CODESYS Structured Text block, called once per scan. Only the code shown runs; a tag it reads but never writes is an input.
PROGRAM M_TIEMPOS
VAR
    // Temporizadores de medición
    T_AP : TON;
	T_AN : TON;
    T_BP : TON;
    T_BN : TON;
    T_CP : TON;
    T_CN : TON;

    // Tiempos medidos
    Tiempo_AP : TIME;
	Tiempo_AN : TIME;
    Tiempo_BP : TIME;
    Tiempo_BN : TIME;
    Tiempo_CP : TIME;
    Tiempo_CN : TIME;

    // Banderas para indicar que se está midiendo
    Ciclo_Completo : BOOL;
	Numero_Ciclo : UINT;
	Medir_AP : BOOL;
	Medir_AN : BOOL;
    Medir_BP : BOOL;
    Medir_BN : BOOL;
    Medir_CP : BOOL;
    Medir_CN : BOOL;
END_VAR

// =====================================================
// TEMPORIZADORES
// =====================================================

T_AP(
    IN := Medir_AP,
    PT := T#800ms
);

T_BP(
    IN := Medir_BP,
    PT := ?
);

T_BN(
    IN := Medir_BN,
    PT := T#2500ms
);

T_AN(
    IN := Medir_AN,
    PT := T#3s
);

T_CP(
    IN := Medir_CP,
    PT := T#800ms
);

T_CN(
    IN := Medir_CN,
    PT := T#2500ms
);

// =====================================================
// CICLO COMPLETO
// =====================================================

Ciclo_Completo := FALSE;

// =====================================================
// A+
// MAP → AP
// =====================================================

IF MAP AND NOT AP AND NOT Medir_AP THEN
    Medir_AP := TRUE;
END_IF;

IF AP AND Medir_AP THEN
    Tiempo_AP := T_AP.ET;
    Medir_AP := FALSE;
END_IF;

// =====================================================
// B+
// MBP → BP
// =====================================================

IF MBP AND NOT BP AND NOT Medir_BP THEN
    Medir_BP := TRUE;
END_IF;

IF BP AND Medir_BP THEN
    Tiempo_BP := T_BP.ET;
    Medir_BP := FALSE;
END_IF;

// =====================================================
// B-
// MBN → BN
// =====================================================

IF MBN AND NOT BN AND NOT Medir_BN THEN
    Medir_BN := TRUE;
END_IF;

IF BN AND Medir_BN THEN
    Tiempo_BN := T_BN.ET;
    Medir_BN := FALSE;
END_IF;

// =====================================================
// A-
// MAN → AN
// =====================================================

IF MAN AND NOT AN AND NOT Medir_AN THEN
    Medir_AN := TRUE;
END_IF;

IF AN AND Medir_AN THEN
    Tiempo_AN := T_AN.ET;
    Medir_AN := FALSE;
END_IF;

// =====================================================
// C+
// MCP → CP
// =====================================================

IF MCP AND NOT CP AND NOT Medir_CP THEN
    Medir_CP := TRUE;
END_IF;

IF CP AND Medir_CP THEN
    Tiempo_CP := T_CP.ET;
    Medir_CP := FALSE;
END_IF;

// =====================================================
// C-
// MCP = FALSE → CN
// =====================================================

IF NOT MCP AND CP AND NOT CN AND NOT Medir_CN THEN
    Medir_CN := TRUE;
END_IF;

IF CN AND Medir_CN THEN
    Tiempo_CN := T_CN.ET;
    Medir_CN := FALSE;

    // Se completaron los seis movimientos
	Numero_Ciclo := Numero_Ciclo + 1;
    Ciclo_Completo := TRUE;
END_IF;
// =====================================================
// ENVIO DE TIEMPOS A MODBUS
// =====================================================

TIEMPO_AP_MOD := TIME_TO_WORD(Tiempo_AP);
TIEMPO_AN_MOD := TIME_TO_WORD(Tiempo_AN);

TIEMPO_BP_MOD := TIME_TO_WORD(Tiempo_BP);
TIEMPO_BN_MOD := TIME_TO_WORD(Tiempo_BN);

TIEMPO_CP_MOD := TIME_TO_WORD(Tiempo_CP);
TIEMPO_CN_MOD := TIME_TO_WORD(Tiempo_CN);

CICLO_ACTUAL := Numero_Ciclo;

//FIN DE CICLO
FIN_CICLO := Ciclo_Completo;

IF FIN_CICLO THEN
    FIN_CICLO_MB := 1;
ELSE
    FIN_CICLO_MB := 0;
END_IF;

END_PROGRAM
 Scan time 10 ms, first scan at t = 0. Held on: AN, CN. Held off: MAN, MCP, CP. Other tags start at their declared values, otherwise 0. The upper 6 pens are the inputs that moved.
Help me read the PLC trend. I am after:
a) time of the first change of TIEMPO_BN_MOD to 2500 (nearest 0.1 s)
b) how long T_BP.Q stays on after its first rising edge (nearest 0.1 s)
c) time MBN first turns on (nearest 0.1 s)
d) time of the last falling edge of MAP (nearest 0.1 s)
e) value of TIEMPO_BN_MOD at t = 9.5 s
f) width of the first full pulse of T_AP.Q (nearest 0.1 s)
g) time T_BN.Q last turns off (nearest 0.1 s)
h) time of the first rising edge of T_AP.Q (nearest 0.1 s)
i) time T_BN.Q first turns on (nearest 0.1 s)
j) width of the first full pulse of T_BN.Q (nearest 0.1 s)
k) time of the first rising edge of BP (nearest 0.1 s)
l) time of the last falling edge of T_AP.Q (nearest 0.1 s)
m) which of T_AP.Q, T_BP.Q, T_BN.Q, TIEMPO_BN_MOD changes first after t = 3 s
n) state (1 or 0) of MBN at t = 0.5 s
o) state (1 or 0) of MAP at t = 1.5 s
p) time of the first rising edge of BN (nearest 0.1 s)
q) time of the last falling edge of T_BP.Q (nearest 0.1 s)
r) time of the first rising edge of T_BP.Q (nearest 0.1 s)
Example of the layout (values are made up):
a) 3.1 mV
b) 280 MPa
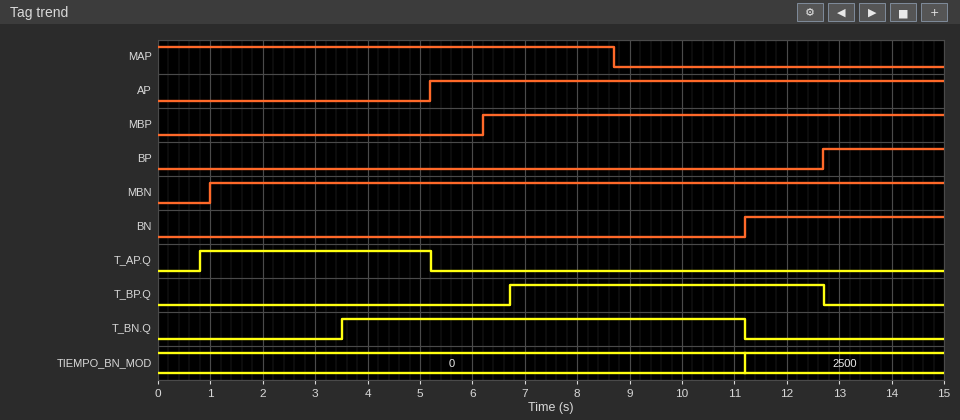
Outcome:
a) 11.2 s
b) 6.0 s
c) 1.0 s
d) 8.7 s
e) 0
f) 4.4 s
g) 11.2 s
h) 0.8 s
i) 3.5 s
j) 7.7 s
k) 12.7 s
l) 5.2 s
m) T_BN.Q
n) 0
o) 1
p) 11.2 s
q) 12.7 s
r) 6.7 s
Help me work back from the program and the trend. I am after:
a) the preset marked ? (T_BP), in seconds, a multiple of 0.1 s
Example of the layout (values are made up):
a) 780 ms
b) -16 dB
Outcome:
a) 0.5 s
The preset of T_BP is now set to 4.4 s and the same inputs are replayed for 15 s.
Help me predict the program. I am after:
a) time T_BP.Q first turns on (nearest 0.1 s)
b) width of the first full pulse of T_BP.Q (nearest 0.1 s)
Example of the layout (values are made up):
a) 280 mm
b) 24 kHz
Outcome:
a) 10.6 s
b) 2.1 s
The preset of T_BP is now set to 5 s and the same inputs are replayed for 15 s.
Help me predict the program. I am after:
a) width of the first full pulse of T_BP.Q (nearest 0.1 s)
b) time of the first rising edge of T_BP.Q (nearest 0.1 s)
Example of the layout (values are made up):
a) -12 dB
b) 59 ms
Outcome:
a) 1.5 s
b) 11.2 s
